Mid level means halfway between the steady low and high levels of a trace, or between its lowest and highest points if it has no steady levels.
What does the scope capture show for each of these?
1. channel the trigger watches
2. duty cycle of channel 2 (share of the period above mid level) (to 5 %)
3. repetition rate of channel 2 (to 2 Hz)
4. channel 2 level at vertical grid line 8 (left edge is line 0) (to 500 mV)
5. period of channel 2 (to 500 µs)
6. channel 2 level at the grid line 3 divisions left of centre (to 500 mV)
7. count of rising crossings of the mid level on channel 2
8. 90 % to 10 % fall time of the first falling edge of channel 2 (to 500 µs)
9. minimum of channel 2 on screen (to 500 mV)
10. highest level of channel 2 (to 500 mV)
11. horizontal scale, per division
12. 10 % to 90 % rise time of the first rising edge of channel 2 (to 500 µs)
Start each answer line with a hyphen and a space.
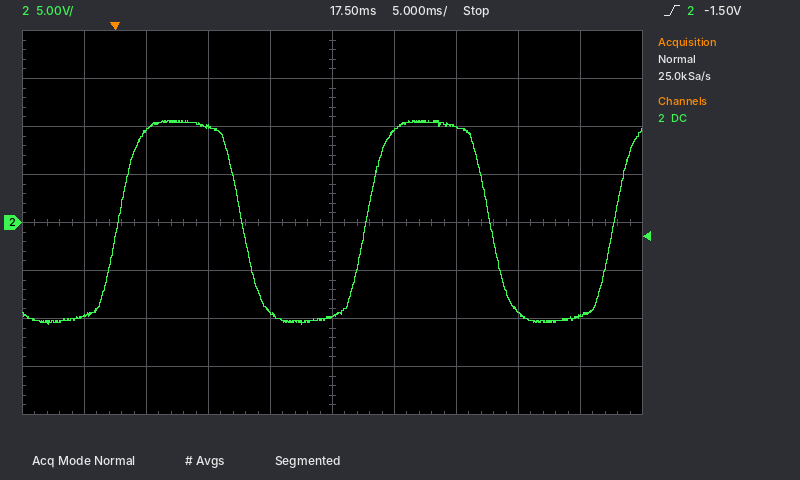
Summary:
- channel 2
- 50 %
- 50 Hz
- -9.5 V
- 20.0 ms
- 9.5 V
- 3
- 3.0 ms
- -10.5 V
- 10.5 V
- 5 ms
- 3.0 ms
